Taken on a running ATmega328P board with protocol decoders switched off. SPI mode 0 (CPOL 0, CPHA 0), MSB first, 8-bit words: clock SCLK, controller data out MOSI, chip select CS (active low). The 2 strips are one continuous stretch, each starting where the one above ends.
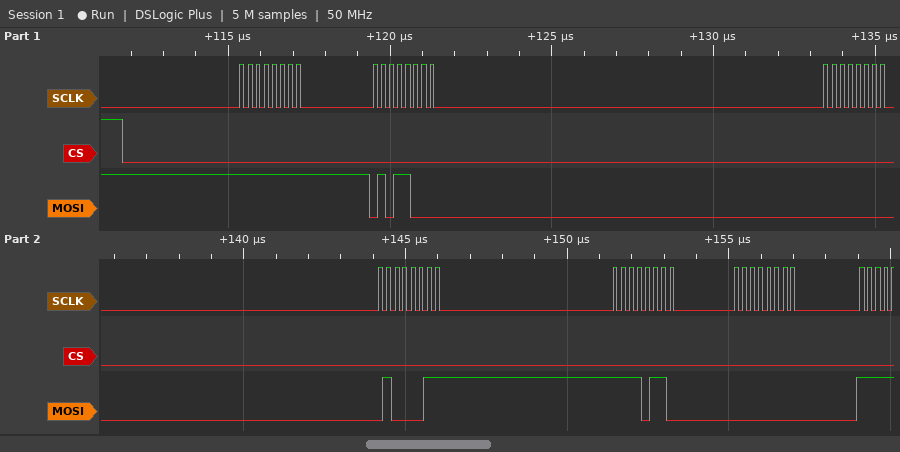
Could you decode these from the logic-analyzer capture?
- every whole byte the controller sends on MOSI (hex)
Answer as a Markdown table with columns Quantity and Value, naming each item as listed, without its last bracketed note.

| Quantity | Value |
|---|---|
| every whole byte the controller sends on MOSI | FF 58 00 43 F6 00 |
